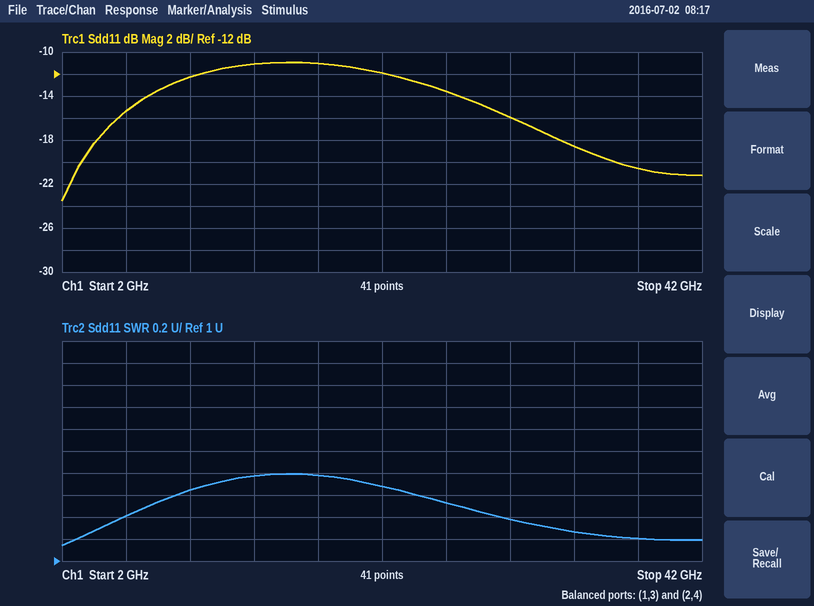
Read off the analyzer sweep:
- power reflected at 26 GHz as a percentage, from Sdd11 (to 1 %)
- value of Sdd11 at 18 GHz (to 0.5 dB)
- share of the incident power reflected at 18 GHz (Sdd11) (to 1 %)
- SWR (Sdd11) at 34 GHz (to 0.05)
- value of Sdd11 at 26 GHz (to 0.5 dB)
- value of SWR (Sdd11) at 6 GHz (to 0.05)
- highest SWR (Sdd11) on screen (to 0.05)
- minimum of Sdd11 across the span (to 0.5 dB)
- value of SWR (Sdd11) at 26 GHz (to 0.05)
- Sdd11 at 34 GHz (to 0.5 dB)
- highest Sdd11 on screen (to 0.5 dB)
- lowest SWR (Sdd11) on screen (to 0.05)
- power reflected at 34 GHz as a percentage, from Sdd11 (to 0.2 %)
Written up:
4 %
-11.0 dB
8 %
1.25
-13.5 dB
1.40
1.80
-23.5 dB
1.55
-18.5 dB
-11.0 dB
1.15
1.4 %
